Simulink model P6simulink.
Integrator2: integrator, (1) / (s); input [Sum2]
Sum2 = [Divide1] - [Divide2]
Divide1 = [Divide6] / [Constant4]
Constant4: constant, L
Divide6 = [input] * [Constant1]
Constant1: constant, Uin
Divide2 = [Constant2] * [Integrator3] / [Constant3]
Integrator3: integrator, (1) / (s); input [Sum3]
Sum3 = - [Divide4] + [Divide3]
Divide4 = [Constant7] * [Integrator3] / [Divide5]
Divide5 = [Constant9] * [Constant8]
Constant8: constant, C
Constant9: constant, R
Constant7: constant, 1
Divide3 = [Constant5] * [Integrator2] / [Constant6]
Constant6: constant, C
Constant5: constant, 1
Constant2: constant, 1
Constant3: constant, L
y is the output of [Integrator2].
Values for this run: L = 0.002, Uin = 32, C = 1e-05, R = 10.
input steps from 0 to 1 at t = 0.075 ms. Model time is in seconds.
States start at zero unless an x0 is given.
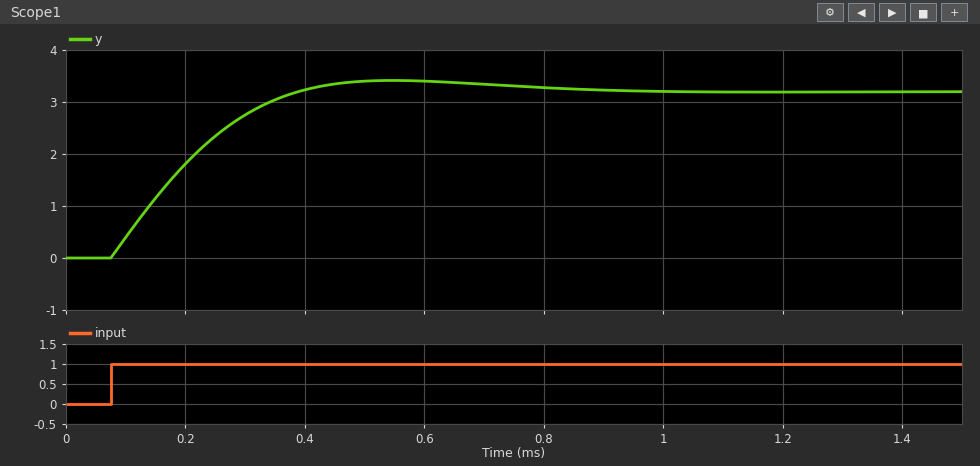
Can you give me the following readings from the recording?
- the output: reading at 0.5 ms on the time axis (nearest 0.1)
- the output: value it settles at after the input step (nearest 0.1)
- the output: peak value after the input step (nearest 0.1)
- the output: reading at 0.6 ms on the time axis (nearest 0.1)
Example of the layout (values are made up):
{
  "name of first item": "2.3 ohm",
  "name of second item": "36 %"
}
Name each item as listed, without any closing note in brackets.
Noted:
{
  "the output: reading at 0.5 ms on the time axis": "3.4",
  "the output: value it settles at after the input step": "3.2",
  "the output: peak value after the input step": "3.4",
  "the output: reading at 0.6 ms on the time axis": "3.4"
}
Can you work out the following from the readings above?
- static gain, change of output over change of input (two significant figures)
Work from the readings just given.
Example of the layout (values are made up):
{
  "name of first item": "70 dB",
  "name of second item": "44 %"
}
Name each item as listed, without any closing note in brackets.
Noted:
{
  "static gain, change of output over change of input": "3.2"
}
